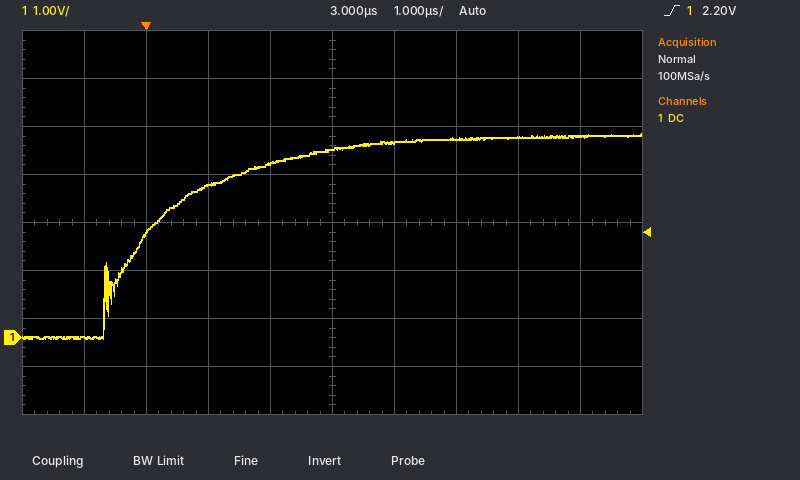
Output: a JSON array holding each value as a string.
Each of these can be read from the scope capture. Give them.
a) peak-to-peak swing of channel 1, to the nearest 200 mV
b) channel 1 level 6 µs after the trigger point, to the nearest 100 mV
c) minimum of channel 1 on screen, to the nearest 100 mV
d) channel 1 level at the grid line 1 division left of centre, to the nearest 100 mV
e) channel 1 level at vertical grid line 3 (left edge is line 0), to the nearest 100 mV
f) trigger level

["4.2 V", "4.2 V", "0.0 V", "3.6 V", "3.2 V", "2.20 V"]
